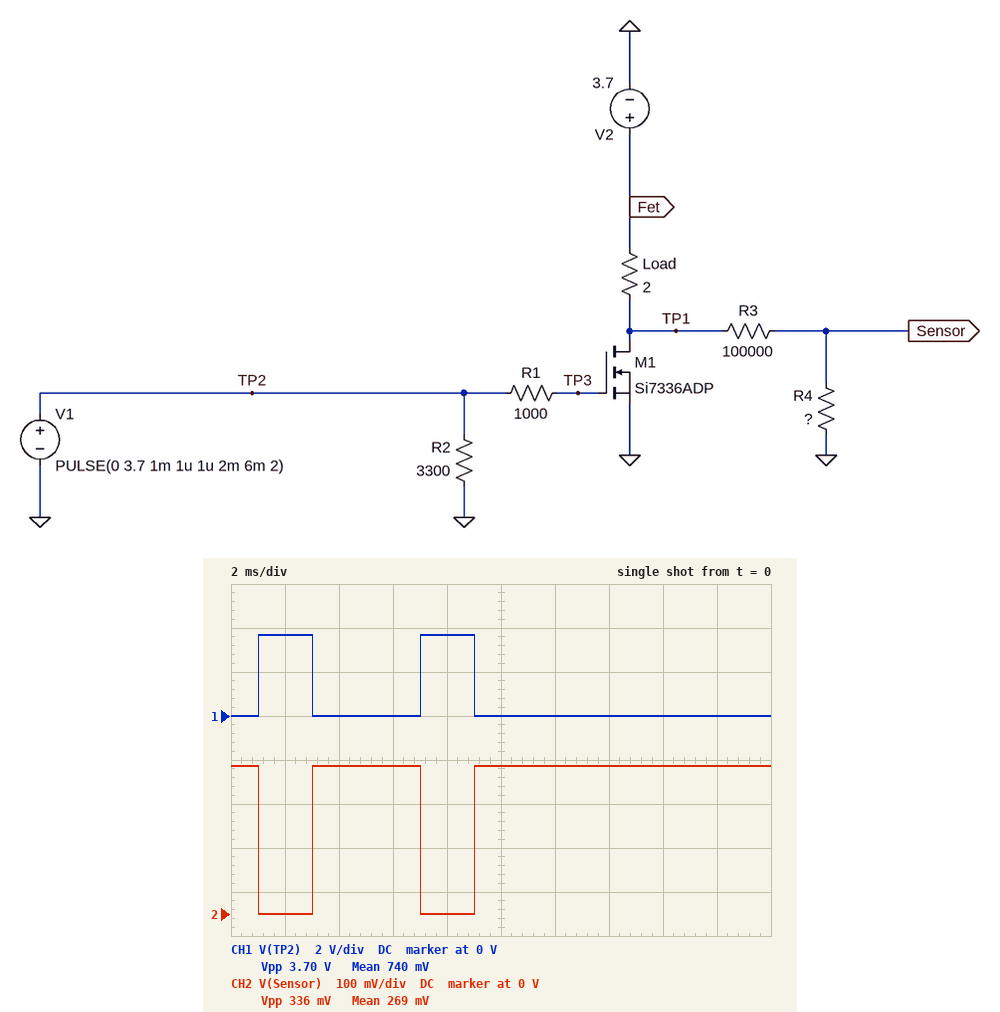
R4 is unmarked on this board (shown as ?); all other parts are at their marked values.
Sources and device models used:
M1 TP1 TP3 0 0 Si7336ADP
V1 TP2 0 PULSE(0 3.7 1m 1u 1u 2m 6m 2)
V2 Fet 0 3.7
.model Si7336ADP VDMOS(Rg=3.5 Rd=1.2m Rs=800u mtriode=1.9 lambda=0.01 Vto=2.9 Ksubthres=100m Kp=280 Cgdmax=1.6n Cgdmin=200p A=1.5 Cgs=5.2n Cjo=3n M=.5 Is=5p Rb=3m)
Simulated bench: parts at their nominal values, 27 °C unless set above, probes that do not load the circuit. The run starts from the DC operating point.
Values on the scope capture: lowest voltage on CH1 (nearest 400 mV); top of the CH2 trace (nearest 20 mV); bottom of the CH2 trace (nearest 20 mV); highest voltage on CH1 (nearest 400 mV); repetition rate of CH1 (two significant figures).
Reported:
0 V
340 mV
0 V
3.6 V
170 Hz
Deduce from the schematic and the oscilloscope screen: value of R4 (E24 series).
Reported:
10 kΩ
